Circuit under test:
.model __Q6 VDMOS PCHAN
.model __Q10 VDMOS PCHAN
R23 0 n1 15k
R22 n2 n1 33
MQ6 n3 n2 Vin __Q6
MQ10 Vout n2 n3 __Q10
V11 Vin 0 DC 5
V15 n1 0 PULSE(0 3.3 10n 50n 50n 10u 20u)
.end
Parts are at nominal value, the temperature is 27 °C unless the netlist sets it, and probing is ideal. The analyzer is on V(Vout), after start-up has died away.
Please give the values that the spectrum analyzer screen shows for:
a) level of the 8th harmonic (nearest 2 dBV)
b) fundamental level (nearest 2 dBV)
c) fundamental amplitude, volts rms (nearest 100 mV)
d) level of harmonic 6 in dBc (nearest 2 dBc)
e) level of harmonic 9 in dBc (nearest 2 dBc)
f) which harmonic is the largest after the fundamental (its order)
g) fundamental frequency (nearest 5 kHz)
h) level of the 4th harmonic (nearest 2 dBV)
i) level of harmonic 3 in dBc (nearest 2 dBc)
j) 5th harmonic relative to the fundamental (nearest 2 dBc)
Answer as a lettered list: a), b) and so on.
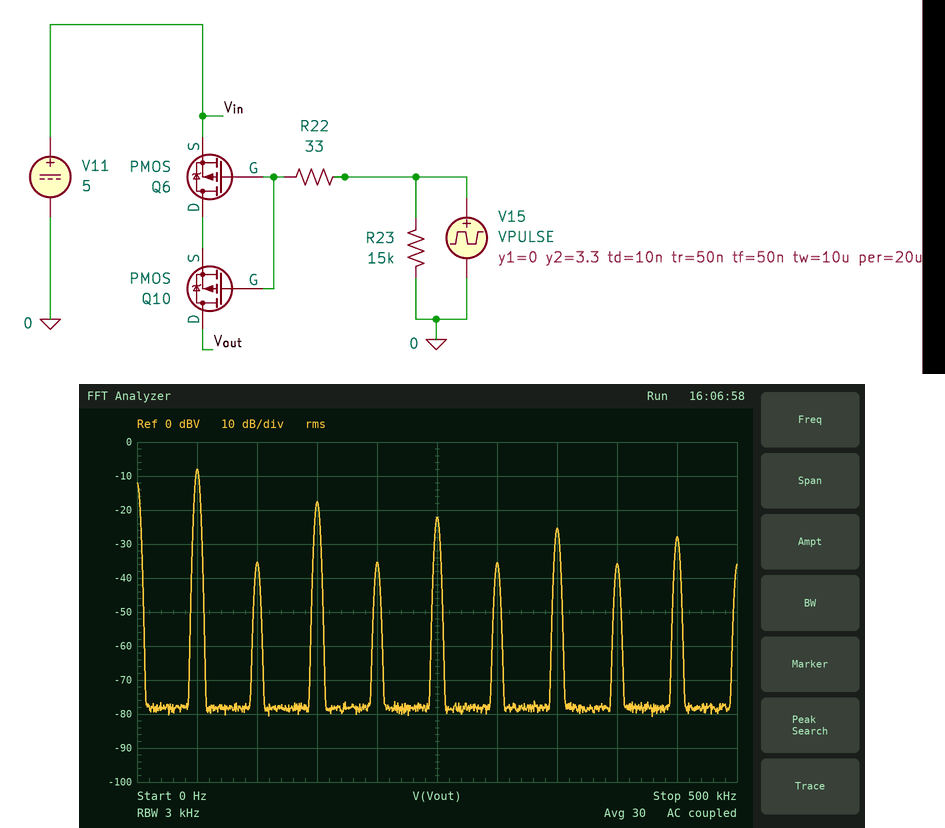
a) -36 dBV
b) -8 dBV
c) 400 mV
d) -28 dBc
e) -20 dBc
f) 3
g) 50 kHz
h) -36 dBV
i) -10 dBc
j) -14 dBc
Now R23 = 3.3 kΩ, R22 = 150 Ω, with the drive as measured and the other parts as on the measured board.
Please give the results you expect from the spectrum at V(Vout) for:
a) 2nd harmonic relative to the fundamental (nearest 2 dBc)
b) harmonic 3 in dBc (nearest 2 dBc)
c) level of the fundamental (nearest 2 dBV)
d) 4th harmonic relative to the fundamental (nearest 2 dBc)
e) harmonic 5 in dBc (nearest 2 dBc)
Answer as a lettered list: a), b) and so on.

a) -14 dBc
b) -12 dBc
c) -8 dBV
d) -14 dBc
e) -20 dBc
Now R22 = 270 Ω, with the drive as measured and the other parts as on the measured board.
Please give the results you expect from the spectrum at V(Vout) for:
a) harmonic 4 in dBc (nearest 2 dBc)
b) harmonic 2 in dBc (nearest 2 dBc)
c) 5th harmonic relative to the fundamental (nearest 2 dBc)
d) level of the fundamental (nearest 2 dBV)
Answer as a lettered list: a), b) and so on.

a) -12 dBc
b) -8 dBc
c) -24 dBc
d) -10 dBV
